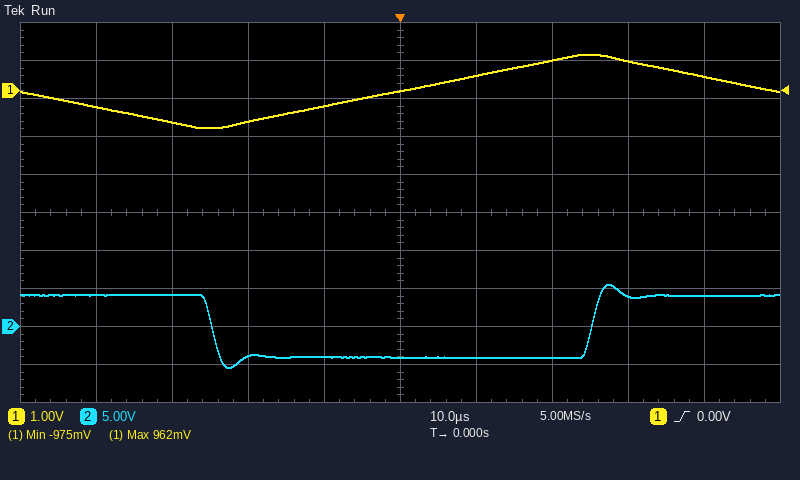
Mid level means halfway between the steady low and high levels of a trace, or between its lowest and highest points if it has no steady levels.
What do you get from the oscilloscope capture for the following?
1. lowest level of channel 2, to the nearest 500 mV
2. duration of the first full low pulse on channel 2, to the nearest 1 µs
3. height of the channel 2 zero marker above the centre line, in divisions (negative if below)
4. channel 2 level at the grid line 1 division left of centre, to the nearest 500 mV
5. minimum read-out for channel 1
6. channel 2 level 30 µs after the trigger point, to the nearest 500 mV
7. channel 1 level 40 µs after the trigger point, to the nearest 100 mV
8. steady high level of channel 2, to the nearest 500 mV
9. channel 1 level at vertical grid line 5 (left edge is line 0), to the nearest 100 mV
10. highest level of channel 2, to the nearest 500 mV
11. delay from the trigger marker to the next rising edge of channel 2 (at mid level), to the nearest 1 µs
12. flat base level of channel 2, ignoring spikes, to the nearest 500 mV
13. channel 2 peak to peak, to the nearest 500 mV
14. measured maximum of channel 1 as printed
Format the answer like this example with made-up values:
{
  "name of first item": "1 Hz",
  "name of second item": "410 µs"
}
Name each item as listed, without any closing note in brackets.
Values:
{
  "lowest level of channel 2, to the nearest 500 mV": "-5.5 V",
  "duration of the first full low pulse on channel 2, to the nearest 1 µs": "50 µs",
  "height of the channel 2 zero marker above the centre line, in divisions": "-3.0 div",
  "channel 2 level at the grid line 1 division left of centre, to the nearest 500 mV": "-4.0 V",
  "minimum read-out for channel 1": "-975 mV",
  "channel 2 level 30 µs after the trigger point, to the nearest 500 mV": "4.0 V",
  "channel 1 level 40 µs after the trigger point, to the nearest 100 mV": "400 mV",
  "steady high level of channel 2, to the nearest 500 mV": "4.0 V",
  "channel 1 level at vertical grid line 5 (left edge is line 0), to the nearest 100 mV": "0.0 V",
  "highest level of channel 2, to the nearest 500 mV": "5.5 V",
  "delay from the trigger marker to the next rising edge of channel 2 (at mid level), to the nearest 1 µs": "25 µs",
  "flat base level of channel 2, ignoring spikes, to the nearest 500 mV": "-4.0 V",
  "channel 2 peak to peak, to the nearest 500 mV": "11.0 V",
  "measured maximum of channel 1 as printed": "962 mV"
}
